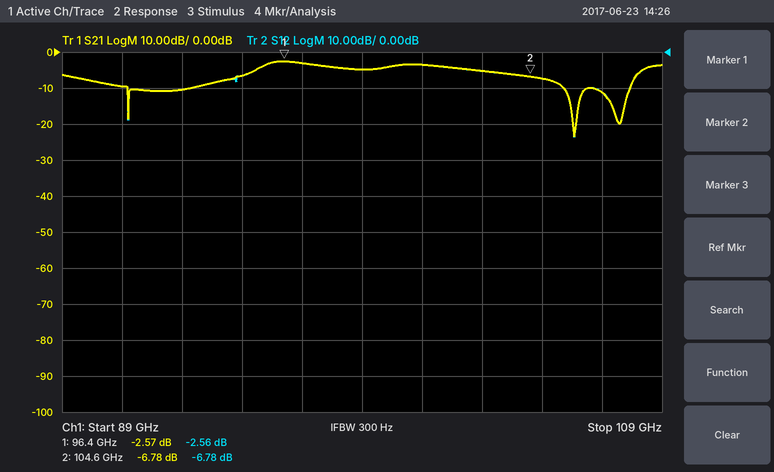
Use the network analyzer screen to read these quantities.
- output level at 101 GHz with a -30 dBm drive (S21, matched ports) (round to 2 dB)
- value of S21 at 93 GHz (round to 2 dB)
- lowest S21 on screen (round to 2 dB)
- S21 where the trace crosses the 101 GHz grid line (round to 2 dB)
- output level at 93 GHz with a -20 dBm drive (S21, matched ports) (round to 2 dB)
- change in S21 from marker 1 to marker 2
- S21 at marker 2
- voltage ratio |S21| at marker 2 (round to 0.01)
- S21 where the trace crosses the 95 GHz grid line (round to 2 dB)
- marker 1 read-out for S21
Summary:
-34 dBm
-10 dB
-24 dB
-4 dB
-30 dBm
-4.21 dB
-6.78 dB
0.46
-6 dB
-2.57 dB
